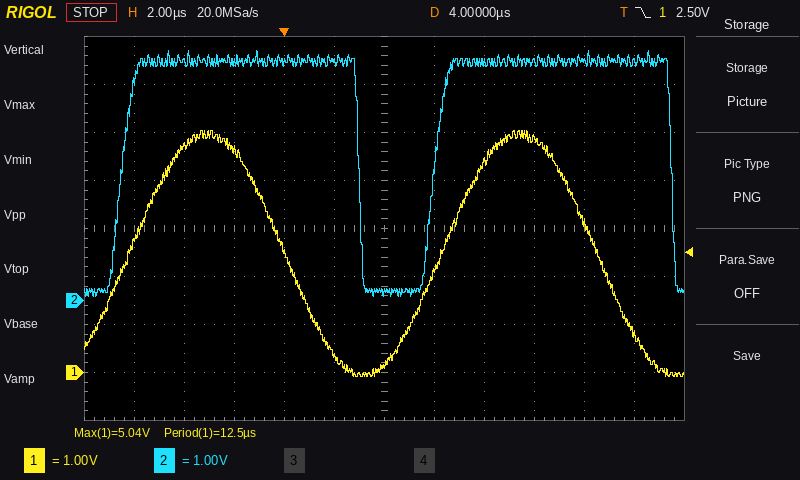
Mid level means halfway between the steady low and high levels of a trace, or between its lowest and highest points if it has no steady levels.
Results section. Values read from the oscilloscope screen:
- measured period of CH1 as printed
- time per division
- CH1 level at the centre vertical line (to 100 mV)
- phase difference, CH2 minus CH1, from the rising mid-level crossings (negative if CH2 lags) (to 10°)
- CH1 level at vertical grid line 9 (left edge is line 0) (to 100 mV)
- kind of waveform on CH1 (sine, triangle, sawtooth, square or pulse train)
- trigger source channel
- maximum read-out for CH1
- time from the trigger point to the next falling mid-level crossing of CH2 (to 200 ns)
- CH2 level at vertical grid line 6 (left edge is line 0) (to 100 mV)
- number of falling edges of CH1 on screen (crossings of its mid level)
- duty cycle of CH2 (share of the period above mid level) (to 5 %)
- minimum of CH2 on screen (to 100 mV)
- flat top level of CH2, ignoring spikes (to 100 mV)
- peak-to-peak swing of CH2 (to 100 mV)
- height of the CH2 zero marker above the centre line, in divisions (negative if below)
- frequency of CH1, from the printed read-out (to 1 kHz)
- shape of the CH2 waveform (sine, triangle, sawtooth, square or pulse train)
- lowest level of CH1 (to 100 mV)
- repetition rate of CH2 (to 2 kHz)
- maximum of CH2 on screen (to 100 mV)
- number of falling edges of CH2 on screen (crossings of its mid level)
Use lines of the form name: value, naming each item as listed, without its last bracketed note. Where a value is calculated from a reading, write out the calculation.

measured period of CH1 as printed: 12.5 µs
time per division: 2 µs
CH1 level at the centre vertical line: 200 mV
phase difference, CH2 minus CH1, from the rising mid-level crossings (negative if CH2 lags): +10°
CH1 level at vertical grid line 9 (left edge is line 0): 4.9 V
kind of waveform on CH1: sine
trigger source channel: CH1
maximum read-out for CH1: 5.04 V
time from the trigger point to the next falling mid-level crossing of CH2: 3.0 µs
CH2 level at vertical grid line 6 (left edge is line 0): 200 mV
number of falling edges of CH1 on screen: 2
duty cycle of CH2 (share of the period above mid level): 75 %
minimum of CH2 on screen: 100 mV
flat top level of CH2, ignoring spikes: 5.0 V
peak-to-peak swing of CH2: 5.2 V − (100 mV) = 5.1 V
height of the CH2 zero marker above the centre line, in divisions: -1.5 div
frequency of CH1, from the printed read-out: 1 / 12.5 µs ≈ 80 kHz
shape of the CH2 waveform: pulse train
lowest level of CH1: -100 mV
repetition rate of CH2: 80 kHz
maximum of CH2 on screen: 5.2 V
number of falling edges of CH2 on screen: 2
